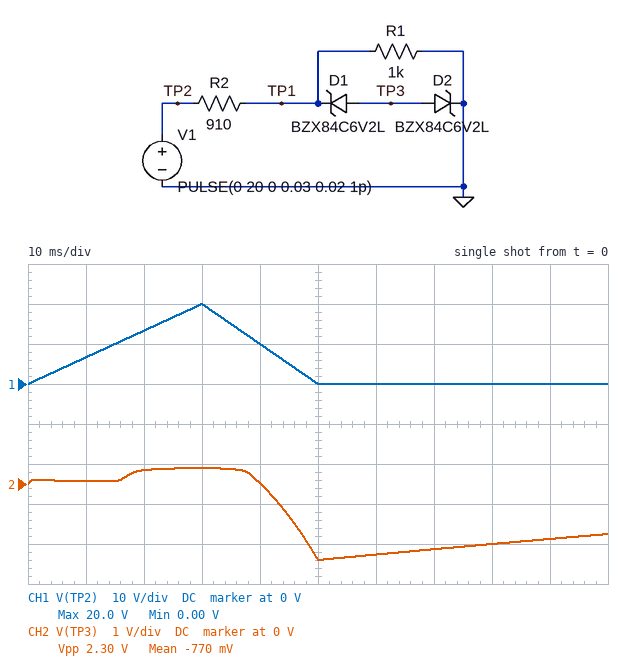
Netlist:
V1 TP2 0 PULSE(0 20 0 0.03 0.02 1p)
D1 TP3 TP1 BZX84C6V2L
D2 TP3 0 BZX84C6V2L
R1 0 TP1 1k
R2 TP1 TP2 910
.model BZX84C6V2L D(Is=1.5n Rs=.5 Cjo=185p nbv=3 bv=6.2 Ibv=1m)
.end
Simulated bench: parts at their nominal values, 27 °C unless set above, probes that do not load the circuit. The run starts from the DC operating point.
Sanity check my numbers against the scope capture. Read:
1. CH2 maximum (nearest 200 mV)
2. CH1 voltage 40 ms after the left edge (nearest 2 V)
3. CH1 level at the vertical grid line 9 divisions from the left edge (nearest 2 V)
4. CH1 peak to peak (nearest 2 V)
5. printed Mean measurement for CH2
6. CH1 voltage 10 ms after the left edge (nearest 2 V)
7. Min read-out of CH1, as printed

400 mV
10 V
0 V
20 V
-770 mV
6 V
0.00 V
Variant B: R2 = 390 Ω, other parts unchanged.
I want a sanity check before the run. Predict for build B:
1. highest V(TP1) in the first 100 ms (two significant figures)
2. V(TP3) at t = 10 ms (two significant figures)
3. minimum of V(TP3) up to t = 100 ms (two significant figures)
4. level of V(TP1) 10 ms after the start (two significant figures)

6.9 V
85 mV
-1.9 V
4.8 V
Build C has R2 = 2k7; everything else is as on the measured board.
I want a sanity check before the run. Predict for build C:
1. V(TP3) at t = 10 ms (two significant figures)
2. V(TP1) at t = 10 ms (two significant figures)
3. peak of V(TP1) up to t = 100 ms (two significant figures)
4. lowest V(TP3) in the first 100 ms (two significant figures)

71 mV
1.8 V
5.4 V
-1.8 V
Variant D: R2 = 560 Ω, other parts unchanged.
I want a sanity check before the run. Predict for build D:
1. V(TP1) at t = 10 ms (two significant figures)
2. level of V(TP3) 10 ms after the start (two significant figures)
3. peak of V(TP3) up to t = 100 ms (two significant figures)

4.3 V
84 mV
430 mV
